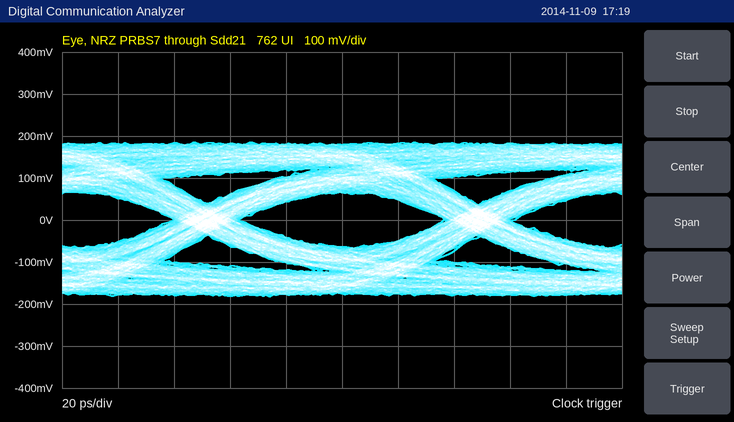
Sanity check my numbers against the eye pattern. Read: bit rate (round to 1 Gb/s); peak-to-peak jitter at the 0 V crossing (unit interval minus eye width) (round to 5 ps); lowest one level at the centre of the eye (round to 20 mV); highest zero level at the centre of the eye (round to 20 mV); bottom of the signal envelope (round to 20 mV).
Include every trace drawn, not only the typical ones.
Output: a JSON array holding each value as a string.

["10 Gb/s", "25 ps", "60 mV", "-60 mV", "-180 mV"]
